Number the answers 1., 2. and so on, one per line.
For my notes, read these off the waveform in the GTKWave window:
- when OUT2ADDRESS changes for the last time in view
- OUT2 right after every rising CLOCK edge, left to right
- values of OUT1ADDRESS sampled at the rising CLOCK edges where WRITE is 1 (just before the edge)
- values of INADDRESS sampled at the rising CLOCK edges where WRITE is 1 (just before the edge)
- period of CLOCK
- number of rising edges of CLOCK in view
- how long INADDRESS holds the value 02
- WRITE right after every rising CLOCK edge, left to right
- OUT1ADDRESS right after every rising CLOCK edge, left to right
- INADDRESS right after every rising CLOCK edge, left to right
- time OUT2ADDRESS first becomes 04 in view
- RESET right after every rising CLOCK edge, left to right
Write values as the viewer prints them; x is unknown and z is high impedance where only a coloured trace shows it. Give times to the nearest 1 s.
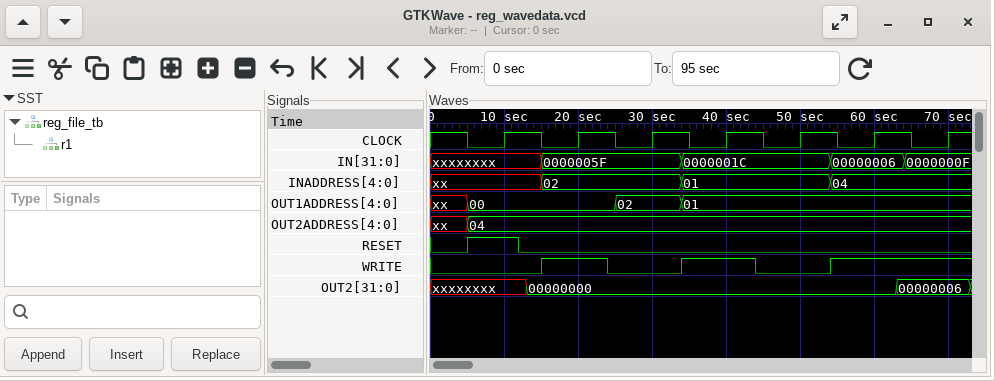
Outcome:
1. 5 s
2. xxxxxxxx, 00000000, 00000000, 00000000, 00000000, 00000000, 00000006
3. 00, 01, 01, 01
4. 02, 01, 04, 04
5. 10 s
6. 7
7. 19 s
8. 0 1 0 1 0 1 1
9. 00, 00, 02, 01, 01, 01, 01
10. xx, 02, 02, 01, 01, 04, 04
11. 5 s
12. 1 0 0 0 0 0 0
